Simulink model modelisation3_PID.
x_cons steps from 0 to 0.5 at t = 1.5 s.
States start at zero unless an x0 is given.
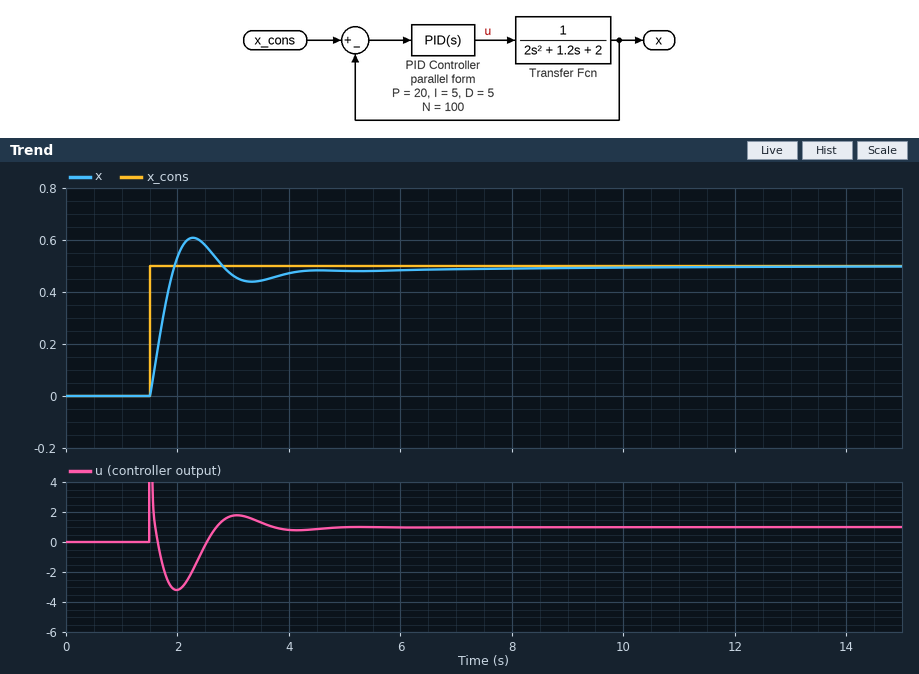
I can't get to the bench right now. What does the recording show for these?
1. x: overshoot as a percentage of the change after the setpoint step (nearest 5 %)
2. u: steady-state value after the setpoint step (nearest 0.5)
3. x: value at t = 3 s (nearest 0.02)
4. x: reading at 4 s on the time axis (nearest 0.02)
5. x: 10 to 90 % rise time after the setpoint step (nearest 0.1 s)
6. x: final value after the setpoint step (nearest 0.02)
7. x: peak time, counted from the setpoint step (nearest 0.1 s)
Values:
20 %
1.0
0.46
0.48
0.3 s
0.50
0.8 s
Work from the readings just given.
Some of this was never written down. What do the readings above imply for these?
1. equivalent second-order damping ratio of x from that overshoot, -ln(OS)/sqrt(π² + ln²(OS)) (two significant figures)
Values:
0.46
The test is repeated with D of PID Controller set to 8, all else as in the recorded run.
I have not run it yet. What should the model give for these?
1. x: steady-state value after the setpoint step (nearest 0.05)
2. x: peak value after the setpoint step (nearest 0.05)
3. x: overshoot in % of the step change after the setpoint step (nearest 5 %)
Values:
0.50
0.55
10 %
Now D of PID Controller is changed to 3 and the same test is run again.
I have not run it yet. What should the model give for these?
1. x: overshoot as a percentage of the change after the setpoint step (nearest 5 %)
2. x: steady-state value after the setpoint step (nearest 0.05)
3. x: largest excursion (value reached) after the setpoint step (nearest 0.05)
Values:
35 %
0.50
0.65
